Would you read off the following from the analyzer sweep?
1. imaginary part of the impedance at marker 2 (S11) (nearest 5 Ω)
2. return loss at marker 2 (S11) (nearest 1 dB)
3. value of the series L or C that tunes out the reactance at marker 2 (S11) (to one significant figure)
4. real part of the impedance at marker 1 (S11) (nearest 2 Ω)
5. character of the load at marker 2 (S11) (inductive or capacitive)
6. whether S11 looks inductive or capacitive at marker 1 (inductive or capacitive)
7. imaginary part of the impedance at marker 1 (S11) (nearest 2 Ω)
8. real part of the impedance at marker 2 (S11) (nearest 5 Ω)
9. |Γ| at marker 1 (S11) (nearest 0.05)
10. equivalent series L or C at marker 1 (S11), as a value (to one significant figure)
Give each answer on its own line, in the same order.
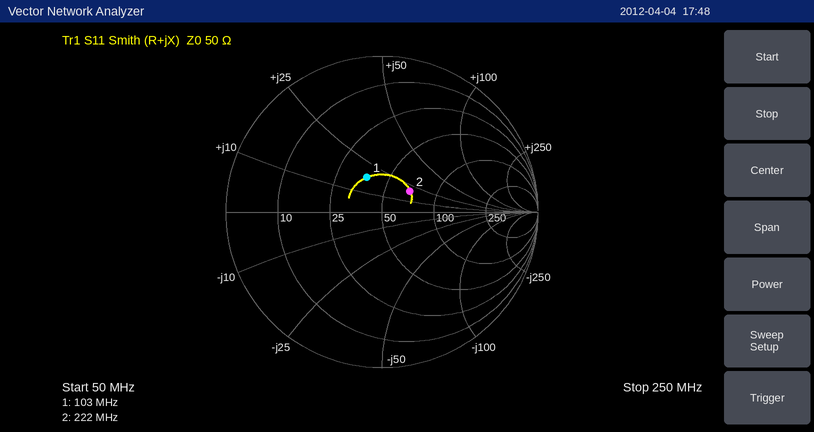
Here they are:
+20 Ω
13 dB
40 pF
38 Ω
inductive
inductive
+18 Ω
70 Ω
0.25
30 nH
